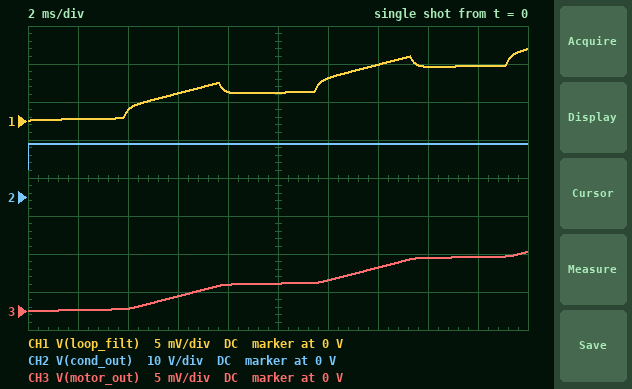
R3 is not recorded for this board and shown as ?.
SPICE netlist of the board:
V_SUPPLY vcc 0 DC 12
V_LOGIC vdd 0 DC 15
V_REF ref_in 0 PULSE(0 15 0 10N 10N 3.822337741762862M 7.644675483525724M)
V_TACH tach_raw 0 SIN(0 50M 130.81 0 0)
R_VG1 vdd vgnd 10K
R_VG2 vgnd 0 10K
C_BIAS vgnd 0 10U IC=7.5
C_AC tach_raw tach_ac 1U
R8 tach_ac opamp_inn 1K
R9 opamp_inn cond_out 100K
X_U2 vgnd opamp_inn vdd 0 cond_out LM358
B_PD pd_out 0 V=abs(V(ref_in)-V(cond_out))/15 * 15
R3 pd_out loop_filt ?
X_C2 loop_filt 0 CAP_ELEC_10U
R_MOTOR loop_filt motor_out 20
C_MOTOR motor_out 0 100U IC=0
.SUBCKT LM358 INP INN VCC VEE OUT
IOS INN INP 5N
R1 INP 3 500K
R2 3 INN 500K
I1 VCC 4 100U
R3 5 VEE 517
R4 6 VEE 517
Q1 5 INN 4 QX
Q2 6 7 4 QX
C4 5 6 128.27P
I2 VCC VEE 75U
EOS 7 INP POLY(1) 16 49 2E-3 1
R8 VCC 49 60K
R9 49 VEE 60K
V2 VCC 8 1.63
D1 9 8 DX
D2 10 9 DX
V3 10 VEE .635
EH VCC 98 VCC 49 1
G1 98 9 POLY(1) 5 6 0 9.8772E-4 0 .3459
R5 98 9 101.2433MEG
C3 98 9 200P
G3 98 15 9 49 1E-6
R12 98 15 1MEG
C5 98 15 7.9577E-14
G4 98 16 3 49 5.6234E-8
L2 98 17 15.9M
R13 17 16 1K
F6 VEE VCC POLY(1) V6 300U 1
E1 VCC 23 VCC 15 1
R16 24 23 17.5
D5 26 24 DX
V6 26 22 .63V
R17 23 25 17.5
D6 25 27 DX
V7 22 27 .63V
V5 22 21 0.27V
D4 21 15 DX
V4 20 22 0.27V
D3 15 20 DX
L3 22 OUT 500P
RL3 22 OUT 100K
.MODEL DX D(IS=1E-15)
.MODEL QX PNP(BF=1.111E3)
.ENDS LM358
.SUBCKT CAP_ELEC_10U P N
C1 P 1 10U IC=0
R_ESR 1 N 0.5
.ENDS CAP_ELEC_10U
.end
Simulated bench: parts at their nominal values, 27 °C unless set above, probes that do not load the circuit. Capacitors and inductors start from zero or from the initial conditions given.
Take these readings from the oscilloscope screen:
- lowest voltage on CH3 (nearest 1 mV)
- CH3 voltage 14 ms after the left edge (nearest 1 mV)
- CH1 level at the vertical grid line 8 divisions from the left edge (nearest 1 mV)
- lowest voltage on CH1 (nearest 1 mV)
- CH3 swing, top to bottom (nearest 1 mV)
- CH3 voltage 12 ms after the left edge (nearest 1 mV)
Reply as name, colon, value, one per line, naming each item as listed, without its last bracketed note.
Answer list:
lowest voltage on CH3: 0 V
CH3 voltage 14 ms after the left edge: 6 mV
CH1 level at the vertical grid line 8 divisions from the left edge: 7 mV
lowest voltage on CH1: 0 V
CH3 swing, top to bottom: 8 mV
CH3 voltage 12 ms after the left edge: 4 mV
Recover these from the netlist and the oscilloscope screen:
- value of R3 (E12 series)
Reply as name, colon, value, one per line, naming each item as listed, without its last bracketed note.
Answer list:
value of R3: 150 kΩ
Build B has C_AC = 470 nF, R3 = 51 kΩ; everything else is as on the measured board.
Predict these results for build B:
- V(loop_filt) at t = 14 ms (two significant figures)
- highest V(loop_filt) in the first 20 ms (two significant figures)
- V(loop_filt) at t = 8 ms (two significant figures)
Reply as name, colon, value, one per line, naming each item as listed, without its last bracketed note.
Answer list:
V(loop_filt) at t = 14 ms: 22 mV
highest V(loop_filt) in the first 20 ms: 28 mV
V(loop_filt) at t = 8 ms: 11 mV
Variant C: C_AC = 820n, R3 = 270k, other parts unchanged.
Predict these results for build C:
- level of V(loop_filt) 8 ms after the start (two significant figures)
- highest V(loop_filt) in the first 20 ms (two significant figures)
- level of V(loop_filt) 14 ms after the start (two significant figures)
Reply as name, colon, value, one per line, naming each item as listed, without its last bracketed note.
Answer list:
level of V(loop_filt) 8 ms after the start: 2.1 mV
highest V(loop_filt) in the first 20 ms: 5.3 mV
level of V(loop_filt) 14 ms after the start: 4.1 mV
